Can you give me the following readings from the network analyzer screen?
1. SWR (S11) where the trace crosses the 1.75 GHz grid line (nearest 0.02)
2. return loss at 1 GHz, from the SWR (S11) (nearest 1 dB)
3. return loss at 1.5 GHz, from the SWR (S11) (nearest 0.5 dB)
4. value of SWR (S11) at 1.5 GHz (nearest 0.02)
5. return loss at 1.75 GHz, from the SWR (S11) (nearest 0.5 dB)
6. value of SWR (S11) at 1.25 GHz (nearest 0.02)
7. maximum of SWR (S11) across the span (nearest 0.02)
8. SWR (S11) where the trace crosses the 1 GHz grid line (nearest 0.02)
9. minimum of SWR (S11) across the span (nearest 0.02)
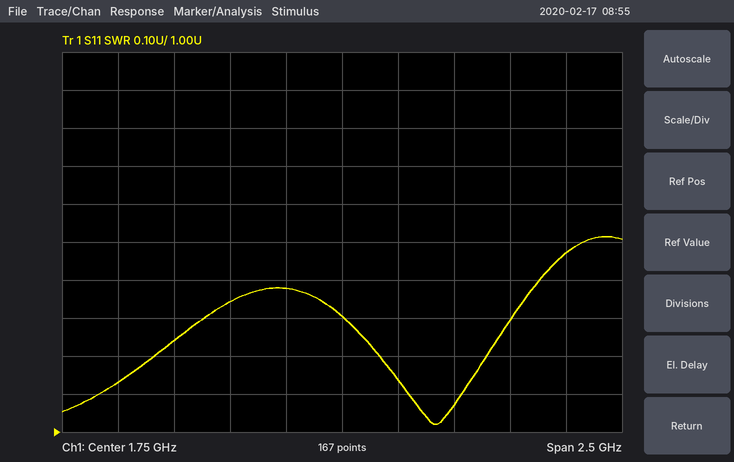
1.30
19 dB
16.0 dB
1.38
17.5 dB
1.34
1.52
1.24
1.02
